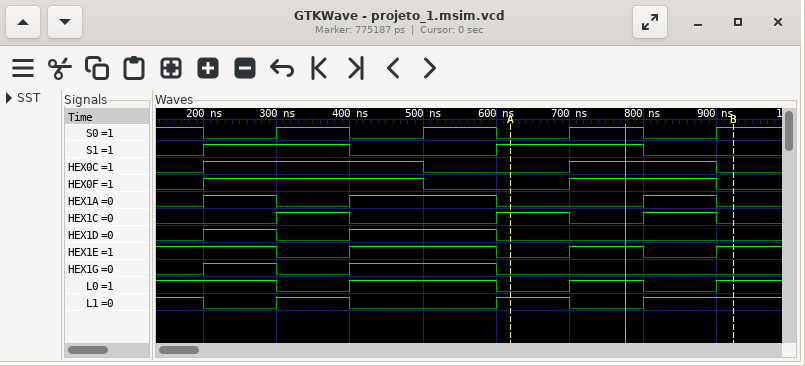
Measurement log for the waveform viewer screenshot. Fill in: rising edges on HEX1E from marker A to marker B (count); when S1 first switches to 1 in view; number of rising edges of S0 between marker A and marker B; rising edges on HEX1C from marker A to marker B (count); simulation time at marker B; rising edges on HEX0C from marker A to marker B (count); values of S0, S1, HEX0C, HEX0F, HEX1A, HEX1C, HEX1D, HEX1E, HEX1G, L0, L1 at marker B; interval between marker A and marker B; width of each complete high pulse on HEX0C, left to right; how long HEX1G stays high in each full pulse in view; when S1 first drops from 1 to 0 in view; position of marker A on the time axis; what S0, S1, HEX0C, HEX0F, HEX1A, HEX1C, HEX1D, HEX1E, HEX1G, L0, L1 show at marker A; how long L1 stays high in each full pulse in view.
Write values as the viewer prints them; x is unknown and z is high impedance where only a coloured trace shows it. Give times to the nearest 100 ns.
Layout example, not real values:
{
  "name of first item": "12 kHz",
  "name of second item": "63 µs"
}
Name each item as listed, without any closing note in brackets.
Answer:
{
  "rising edges on HEX1E from marker A to marker B": "2",
  "when S1 first switches to 1 in view": "200 ns",
  "number of rising edges of S0 between marker A and marker B": "2",
  "rising edges on HEX1C from marker A to marker B": "1",
  "simulation time at marker B": "900 ns",
  "rising edges on HEX0C from marker A to marker B": "1",
  "values of S0, S1, HEX0C, HEX0F, HEX1A, HEX1C, HEX1D, HEX1E, HEX1G, L0, L1 at marker B": "S0=1, S1=0, HEX0C=0, HEX0F=0, HEX1A=0, HEX1C=0, HEX1D=0, HEX1E=1, HEX1G=0, L0=1, L1=1",
  "interval between marker A and marker B": "300 ns",
  "width of each complete high pulse on HEX0C, left to right": "300 ns, 200 ns",
  "how long HEX1G stays high in each full pulse in view": "100 ns, 200 ns",
  "when S1 first drops from 1 to 0 in view": "400 ns",
  "position of marker A on the time axis": "600 ns",
  "what S0, S1, HEX0C, HEX0F, HEX1A, HEX1C, HEX1D, HEX1E, HEX1G, L0, L1 show at marker A": "S0=0, S1=1, HEX0C=0, HEX0F=0, HEX1A=0, HEX1C=1, HEX1D=0, HEX1E=0, HEX1G=0, L0=0, L1=1",
  "how long L1 stays high in each full pulse in view": "100 ns, 100 ns"
}
